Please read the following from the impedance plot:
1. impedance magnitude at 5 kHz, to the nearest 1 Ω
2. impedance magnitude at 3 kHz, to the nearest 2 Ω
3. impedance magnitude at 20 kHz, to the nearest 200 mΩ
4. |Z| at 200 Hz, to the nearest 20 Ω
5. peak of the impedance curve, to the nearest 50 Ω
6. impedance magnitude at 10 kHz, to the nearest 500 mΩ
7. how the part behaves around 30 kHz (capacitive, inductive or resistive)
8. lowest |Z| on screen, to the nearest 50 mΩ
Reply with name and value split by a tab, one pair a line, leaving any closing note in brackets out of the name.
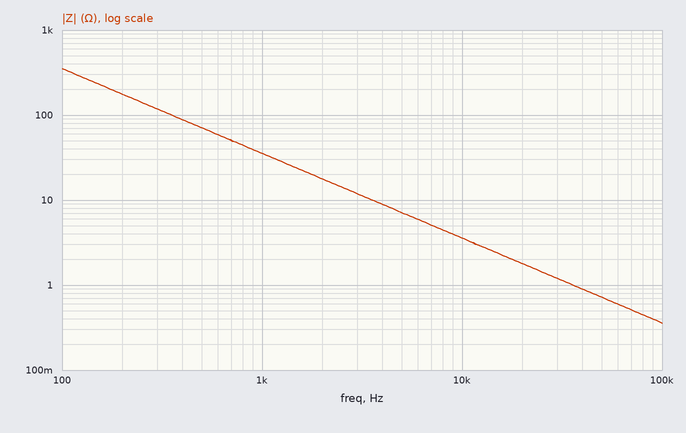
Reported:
impedance magnitude at 5 kHz, to the nearest 1 Ω	7 Ω
impedance magnitude at 3 kHz, to the nearest 2 Ω	12 Ω
impedance magnitude at 20 kHz, to the nearest 200 mΩ	1.8 Ω
|Z| at 200 Hz, to the nearest 20 Ω	180 Ω
peak of the impedance curve, to the nearest 50 Ω	350 Ω
impedance magnitude at 10 kHz, to the nearest 500 mΩ	3.5 Ω
how the part behaves around 30 kHz	capacitive
lowest |Z| on screen, to the nearest 50 mΩ	350 mΩ
